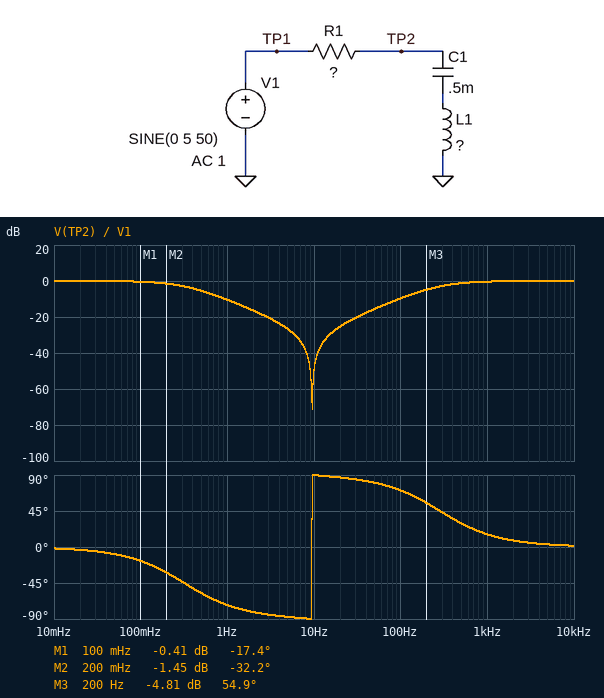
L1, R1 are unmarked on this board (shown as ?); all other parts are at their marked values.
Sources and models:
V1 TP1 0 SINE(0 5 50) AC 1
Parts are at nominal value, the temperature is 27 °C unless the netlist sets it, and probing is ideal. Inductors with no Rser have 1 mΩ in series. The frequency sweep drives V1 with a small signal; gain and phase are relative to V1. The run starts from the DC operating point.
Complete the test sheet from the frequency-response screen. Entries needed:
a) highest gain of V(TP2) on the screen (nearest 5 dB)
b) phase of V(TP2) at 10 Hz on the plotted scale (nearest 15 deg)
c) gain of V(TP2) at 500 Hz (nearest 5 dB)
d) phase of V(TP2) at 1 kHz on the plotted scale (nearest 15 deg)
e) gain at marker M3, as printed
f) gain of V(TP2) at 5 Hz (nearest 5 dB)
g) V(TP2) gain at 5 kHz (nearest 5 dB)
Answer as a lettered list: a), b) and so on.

a) 0 dB
b) 90 deg
c) 0 dB
d) 15 deg
e) -4.81 dB
f) -25 dB
g) 0 dB
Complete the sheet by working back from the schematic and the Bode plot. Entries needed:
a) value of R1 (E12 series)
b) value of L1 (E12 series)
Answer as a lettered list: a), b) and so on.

a) 1 kΩ
b) 560 mH
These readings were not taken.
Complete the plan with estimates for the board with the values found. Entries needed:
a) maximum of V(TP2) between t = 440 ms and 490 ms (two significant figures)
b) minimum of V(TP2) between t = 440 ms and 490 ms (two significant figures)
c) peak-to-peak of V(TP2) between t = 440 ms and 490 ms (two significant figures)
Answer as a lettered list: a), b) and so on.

a) 850 mV
b) -820 mV
c) 1.7 V
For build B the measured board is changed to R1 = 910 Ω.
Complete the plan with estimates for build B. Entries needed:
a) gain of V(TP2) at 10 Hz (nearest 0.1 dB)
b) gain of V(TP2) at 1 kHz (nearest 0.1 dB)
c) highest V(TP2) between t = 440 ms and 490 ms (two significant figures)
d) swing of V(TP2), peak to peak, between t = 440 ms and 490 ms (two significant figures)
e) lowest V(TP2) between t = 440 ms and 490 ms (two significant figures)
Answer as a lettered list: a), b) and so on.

a) -48.7 dB
b) -0.3 dB
c) 930 mV
d) 1.8 V
e) -900 mV
